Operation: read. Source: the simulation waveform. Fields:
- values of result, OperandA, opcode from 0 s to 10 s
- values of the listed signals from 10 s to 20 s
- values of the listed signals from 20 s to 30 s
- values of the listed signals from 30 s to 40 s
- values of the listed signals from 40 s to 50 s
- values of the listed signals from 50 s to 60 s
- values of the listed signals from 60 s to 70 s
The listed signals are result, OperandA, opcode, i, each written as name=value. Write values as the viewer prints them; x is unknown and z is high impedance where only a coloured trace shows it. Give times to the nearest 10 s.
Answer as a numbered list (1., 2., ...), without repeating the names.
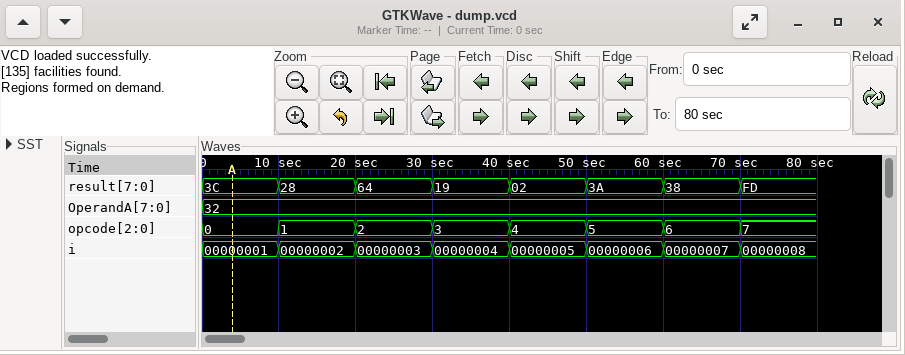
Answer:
1. result=3C, OperandA=32, opcode=0
2. result=28, OperandA=32, opcode=1, i=00000002
3. result=64, OperandA=32, opcode=2, i=00000003
4. result=19, OperandA=32, opcode=3, i=00000004
5. result=02, OperandA=32, opcode=4, i=00000005
6. result=3A, OperandA=32, opcode=5, i=00000006
7. result=38, OperandA=32, opcode=6, i=00000007
